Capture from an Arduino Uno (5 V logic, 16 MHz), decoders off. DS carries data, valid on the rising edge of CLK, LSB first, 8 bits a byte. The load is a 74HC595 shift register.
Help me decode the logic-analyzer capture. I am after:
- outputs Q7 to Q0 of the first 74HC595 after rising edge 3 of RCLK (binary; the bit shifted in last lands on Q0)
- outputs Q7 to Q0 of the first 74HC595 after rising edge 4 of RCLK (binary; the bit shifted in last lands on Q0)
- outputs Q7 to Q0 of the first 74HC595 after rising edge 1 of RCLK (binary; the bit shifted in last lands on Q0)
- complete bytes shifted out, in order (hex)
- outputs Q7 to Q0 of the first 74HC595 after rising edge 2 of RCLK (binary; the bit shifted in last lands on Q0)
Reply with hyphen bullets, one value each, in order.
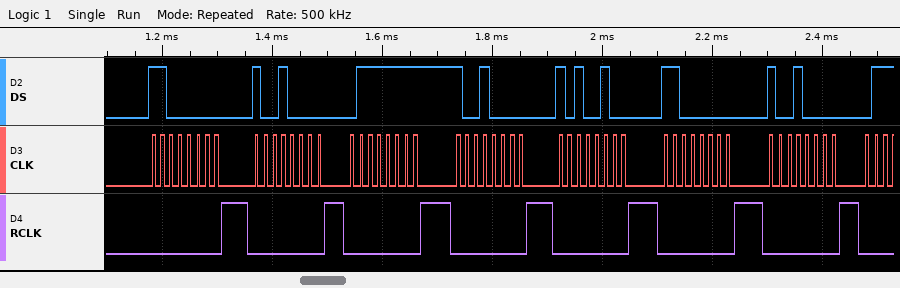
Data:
- 01111111
- 10010000
- 11000000
- 03 09 FE 09 25 03 09
- 10010000
